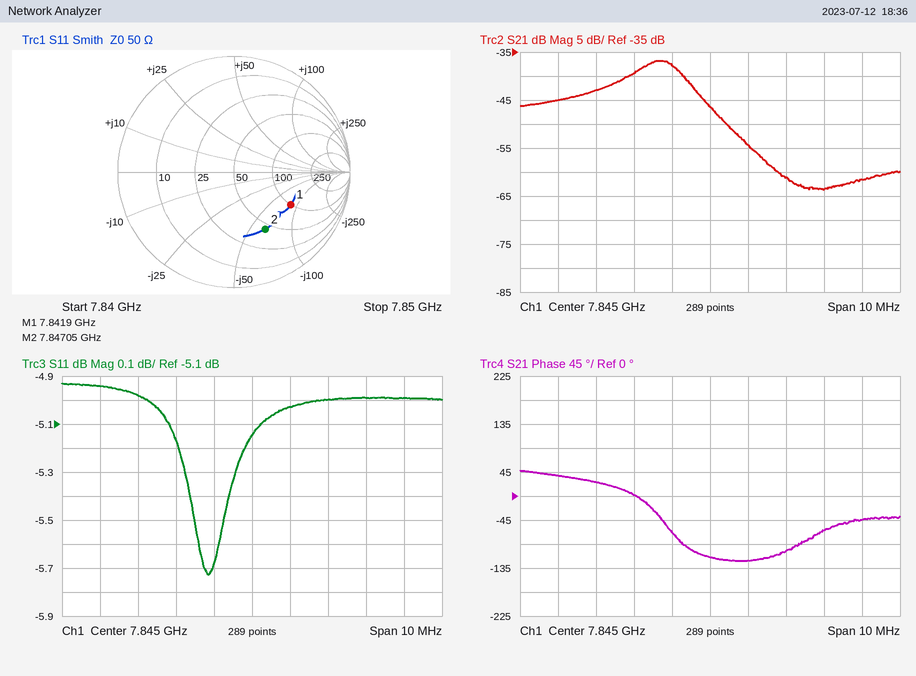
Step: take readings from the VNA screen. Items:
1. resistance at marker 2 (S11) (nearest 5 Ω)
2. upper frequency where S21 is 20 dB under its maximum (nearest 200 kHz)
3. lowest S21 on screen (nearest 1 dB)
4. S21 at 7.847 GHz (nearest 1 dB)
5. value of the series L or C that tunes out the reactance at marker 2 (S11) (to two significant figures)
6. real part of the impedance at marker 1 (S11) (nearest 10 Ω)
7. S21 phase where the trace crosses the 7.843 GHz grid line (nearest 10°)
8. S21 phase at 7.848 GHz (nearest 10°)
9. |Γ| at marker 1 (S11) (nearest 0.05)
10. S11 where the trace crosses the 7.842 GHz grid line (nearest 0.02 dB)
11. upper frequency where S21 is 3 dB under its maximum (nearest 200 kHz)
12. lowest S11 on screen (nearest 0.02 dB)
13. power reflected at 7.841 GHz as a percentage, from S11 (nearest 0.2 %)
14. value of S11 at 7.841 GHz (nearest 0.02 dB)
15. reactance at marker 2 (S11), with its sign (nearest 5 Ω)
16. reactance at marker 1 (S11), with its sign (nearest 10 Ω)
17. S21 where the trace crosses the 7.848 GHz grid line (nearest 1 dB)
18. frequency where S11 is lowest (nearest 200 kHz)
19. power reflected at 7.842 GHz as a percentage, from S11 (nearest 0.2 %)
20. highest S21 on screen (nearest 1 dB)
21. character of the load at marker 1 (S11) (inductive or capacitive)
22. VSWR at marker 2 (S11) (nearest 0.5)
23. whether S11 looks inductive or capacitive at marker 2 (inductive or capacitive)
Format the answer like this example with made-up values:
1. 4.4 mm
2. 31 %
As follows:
1. 45 Ω
2. 7.8464 GHz
3. -64 dB
4. -61 dB
5. 1.3 nH
6. 100 Ω
7. 0°
8. -60°
9. 0.55
10. -4.98 dB
11. 7.8442 GHz
12. -5.72 dB
13. 32.0 %
14. -4.94 dB
15. -65 Ω
16. -80 Ω
17. -64 dB
18. 7.8438 GHz
19. 31.8 %
20. -37 dB
21. capacitive
22. 3.5
23. capacitive
